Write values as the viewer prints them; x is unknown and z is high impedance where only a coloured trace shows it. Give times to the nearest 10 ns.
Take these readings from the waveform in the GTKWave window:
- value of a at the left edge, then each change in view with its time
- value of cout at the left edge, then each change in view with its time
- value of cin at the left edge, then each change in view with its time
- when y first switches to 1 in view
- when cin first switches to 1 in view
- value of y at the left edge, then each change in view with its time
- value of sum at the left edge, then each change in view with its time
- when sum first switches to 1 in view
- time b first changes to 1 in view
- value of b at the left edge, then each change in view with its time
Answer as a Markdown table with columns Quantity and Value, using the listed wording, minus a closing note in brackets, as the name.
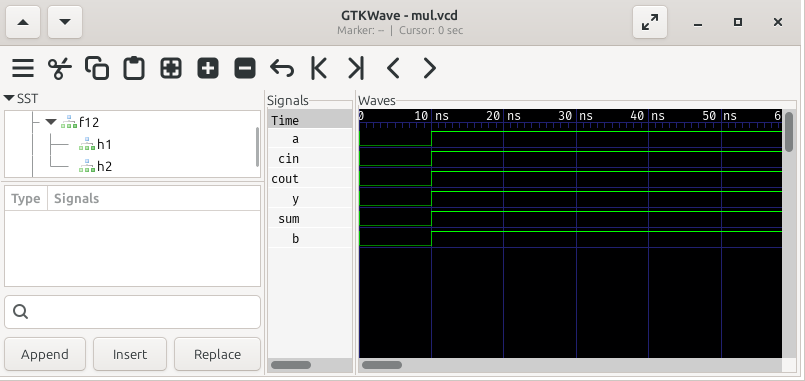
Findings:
| Quantity | Value |
|---|---|
| value of a at the left edge, then each change in view with its time | 0, 1 at 10 ns |
| value of cout at the left edge, then each change in view with its time | 0, 1 at 10 ns |
| value of cin at the left edge, then each change in view with its time | 0, 1 at 10 ns |
| when y first switches to 1 in view | 10 ns |
| when cin first switches to 1 in view | 10 ns |
| value of y at the left edge, then each change in view with its time | 0, 1 at 10 ns |
| value of sum at the left edge, then each change in view with its time | 0, 1 at 10 ns |
| when sum first switches to 1 in view | 10 ns |
| time b first changes to 1 in view | 10 ns |
| value of b at the left edge, then each change in view with its time | 0, 1 at 10 ns |
